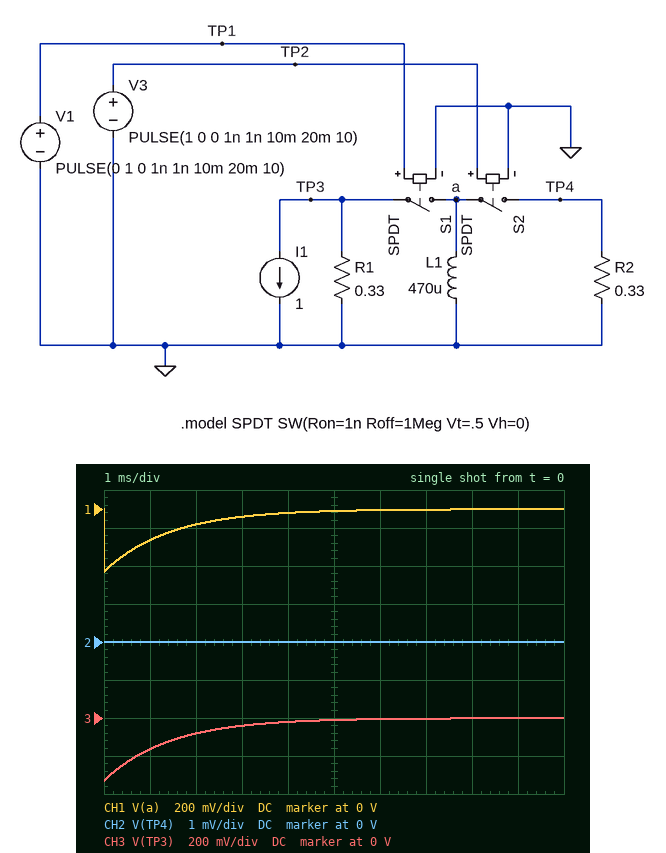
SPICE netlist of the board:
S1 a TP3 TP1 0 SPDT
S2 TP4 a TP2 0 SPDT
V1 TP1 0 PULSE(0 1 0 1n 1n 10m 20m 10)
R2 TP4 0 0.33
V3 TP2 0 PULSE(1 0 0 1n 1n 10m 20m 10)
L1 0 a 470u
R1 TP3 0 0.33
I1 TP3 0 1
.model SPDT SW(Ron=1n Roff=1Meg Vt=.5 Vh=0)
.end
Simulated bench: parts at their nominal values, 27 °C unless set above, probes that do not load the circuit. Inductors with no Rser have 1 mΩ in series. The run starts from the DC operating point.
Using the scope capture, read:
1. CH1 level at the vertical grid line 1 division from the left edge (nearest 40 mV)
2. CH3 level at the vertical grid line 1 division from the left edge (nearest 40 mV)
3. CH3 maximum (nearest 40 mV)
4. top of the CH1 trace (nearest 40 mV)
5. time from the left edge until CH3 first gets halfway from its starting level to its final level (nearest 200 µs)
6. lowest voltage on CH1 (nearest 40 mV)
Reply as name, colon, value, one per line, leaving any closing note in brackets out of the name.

CH1 level at the vertical grid line 1 division from the left edge: -160 mV
CH3 level at the vertical grid line 1 division from the left edge: -160 mV
CH3 maximum: 0 V
top of the CH1 trace: 0 V
time from the left edge until CH3 first gets halfway from its starting level to its final level: 1.0 ms
lowest voltage on CH1: -320 mV
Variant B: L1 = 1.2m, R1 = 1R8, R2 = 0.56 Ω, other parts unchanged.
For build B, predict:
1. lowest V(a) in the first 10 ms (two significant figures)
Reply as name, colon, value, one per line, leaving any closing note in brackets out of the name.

lowest V(a) in the first 10 ms: -1.8 V
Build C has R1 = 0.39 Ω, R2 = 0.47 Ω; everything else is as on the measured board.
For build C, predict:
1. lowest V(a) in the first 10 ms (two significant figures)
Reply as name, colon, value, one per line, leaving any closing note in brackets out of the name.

lowest V(a) in the first 10 ms: -390 mV
